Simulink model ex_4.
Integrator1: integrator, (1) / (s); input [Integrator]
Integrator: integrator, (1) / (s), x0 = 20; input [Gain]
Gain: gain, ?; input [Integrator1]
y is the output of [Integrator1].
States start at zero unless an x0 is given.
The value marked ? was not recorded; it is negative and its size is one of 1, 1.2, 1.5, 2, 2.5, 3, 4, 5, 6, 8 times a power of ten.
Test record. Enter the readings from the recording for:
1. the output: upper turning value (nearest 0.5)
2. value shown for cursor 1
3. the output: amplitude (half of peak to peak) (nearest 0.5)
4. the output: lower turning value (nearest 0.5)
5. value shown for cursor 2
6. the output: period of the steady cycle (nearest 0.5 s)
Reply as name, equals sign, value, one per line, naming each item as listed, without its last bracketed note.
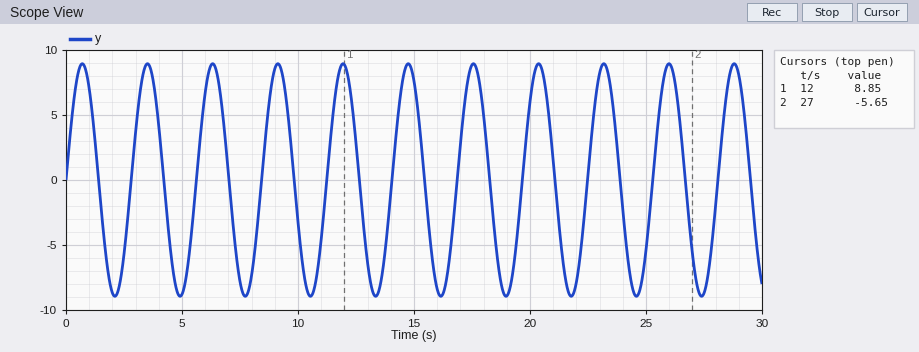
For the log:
the output: upper turning value = 9.0
value shown for cursor 1 = 8.85
the output: amplitude (half of peak to peak) = 9.0
the output: lower turning value = -9.0
value shown for cursor 2 = -5.65
the output: period of the steady cycle = 3.0 s
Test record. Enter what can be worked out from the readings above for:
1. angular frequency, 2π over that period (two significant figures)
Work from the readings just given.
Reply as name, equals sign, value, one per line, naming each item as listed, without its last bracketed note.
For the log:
angular frequency, 2π over that period = 2.1 rad/s
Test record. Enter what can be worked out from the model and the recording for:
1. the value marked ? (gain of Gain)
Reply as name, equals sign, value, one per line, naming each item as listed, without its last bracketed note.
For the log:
the value marked ? = -5
